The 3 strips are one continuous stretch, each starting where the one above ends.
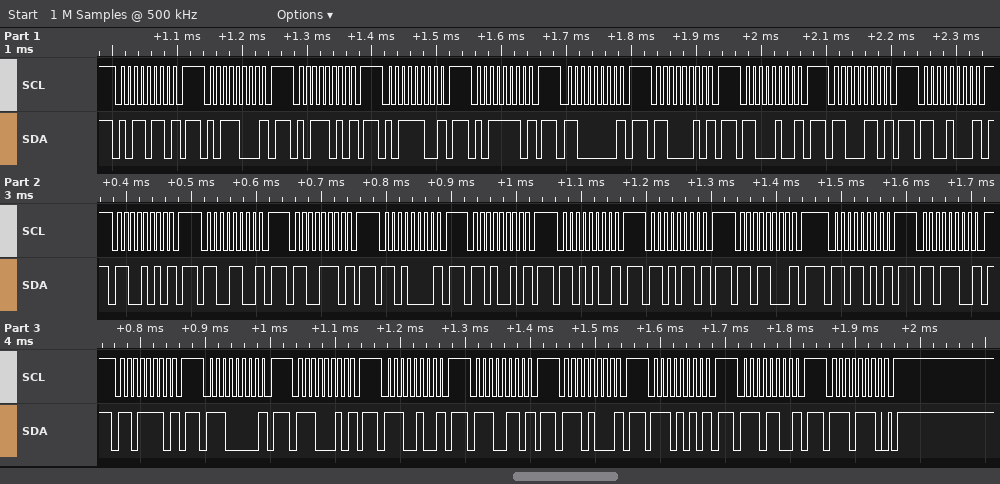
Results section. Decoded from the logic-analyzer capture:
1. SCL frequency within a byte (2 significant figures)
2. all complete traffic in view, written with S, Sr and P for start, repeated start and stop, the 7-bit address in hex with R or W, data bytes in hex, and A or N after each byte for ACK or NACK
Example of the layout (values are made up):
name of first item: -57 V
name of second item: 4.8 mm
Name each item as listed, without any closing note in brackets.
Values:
SCL frequency within a byte: 100 kHz
all complete traffic in view, written with S, Sr and P for start, repeated start and stop, the 7-bit address in hex with R or W, data bytes in hex, and A or N after each byte for ACK or NACK: S 5BW N P S 5CW N P S 5DW N P S 5EW N P S 5FW N P S 60W N P S 61W N P S 62W N P S 63W N P S 64W N P S 65W N P S 66W N P S 67W N P S 68W N P S 69W N P S 6AW N P S 6BW N P S 6CW N P S 6DW N P S 6EW N P S 6FW N P S 70W N P S 71W N P S 72W N P S 73W N P S 74W N P S 75W N P S 76W N P S 77W A P
